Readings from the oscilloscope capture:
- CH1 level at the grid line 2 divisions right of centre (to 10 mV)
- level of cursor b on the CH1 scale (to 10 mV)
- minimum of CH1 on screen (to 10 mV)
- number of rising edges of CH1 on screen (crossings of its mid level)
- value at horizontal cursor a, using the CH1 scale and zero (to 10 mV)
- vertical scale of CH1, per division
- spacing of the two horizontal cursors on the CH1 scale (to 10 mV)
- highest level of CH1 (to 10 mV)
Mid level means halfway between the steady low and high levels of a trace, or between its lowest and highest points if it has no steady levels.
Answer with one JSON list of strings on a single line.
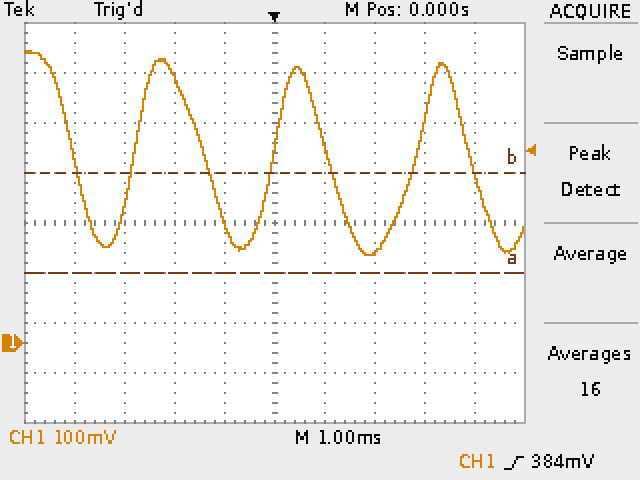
["180 mV", "340 mV", "180 mV", "3", "140 mV", "100 mV", "200 mV", "580 mV"]
